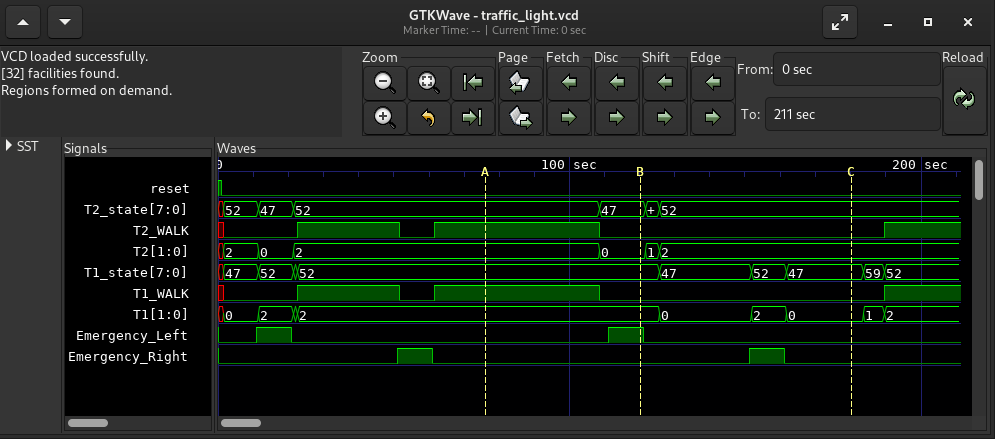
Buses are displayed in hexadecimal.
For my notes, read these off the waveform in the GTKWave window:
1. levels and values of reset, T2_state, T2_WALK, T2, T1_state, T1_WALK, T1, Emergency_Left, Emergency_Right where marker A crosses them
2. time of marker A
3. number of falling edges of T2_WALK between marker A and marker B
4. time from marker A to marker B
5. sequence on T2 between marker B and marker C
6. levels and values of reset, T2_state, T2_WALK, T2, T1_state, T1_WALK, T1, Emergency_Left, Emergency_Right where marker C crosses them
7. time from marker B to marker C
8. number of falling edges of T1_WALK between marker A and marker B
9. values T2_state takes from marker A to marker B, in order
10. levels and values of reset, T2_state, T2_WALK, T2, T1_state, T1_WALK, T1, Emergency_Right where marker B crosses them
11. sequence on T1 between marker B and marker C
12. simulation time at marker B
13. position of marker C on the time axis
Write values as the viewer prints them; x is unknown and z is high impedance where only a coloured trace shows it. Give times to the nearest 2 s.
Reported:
reset=0, T2_state=52, T2_WALK=1, T2=2, T1_state=52, T1_WALK=1, T1=2, Emergency_Left=0, Emergency_Right=0
76 s
1
44 s
0, 1, 2
reset=0, T2_state=52, T2_WALK=0, T2=2, T1_state=47, T1_WALK=0, T1=0, Emergency_Left=0, Emergency_Right=0
60 s
1
52, 47
reset=0, T2_state=47, T2_WALK=0, T2=0, T1_state=52, T1_WALK=0, T1=2, Emergency_Right=0
2, 0, 2, 0
120 s
180 s
